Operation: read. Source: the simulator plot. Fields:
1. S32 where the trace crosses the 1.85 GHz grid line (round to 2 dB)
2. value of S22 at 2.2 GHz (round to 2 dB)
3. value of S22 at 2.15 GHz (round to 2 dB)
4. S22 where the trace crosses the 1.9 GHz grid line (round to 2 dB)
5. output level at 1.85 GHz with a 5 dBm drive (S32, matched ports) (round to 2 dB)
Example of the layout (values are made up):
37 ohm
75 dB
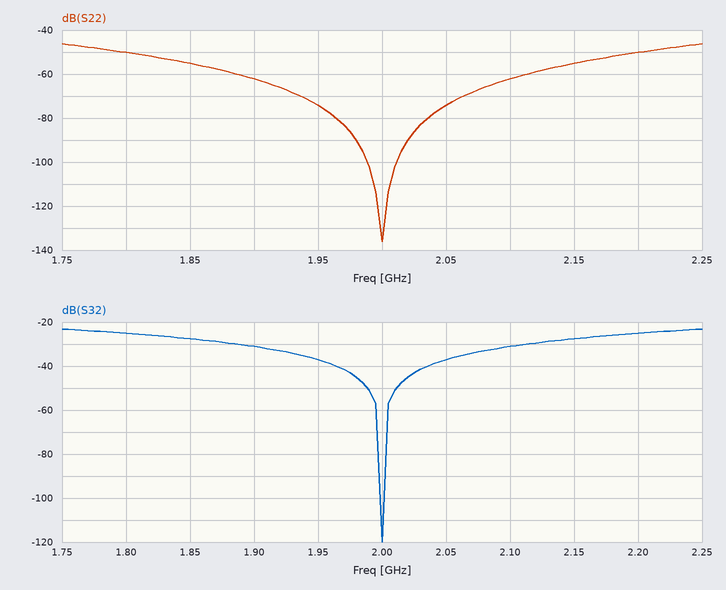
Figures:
-28 dB
-50 dB
-56 dB
-62 dB
-22 dBm
